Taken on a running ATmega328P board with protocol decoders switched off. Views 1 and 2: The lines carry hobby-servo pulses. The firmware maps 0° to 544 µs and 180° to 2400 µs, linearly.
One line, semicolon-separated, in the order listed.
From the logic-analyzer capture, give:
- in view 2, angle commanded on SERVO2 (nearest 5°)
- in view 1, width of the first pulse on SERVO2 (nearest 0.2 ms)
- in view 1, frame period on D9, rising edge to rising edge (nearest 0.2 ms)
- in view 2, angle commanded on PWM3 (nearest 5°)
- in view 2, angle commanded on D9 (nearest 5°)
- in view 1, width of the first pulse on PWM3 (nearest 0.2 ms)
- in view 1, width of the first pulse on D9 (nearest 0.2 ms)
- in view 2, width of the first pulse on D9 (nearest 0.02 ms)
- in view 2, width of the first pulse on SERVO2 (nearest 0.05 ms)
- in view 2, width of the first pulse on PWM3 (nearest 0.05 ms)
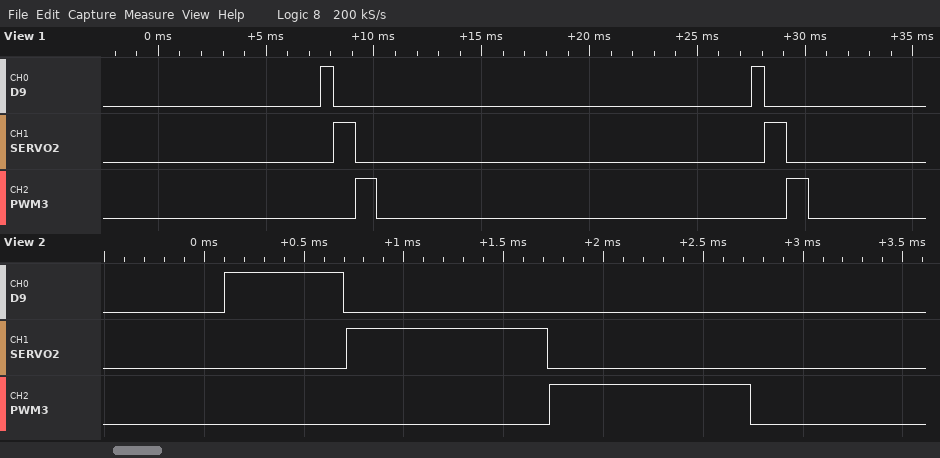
45°; 1.0 ms; 20.0 ms; 45°; 5°; 1.0 ms; 0.6 ms; 0.60 ms; 1.00 ms; 1.00 ms
